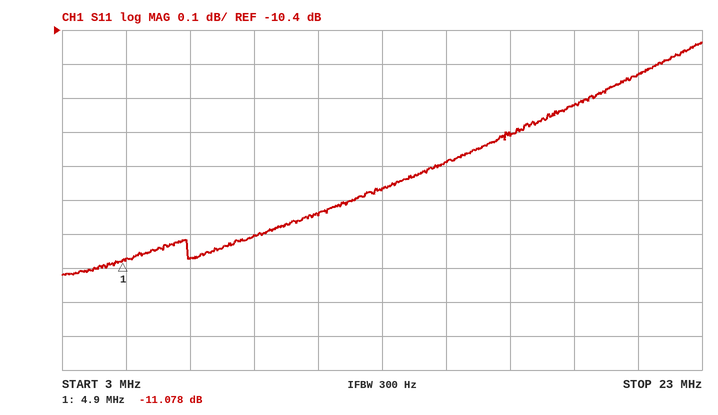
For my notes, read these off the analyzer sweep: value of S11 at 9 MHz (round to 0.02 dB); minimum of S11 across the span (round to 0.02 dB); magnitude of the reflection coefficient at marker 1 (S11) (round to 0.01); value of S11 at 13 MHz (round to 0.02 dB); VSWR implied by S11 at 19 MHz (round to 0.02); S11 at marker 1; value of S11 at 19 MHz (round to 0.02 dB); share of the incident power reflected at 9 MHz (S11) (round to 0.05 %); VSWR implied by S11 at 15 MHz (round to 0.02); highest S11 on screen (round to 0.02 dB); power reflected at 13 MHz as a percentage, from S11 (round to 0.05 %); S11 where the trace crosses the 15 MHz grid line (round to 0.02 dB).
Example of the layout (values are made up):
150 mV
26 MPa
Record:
-11.00 dB
-11.12 dB
0.28
-10.86 dB
1.84
-11.078 dB
-10.62 dB
7.95 %
1.82
-10.44 dB
8.20 %
-10.78 dB
